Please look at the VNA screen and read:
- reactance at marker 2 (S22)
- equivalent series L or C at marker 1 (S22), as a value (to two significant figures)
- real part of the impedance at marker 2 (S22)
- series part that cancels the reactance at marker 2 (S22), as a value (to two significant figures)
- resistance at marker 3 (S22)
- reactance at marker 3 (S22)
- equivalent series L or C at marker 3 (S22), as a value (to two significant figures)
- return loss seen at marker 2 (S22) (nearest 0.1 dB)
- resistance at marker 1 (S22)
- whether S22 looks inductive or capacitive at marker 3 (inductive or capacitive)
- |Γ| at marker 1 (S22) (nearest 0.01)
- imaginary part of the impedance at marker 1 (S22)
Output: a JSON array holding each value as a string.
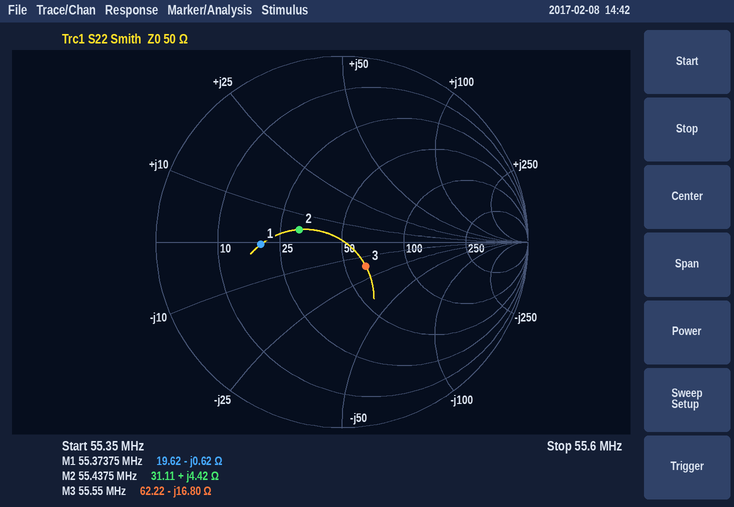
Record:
["+4.42 Ω", "4.6 nF", "31.11 Ω", "650 pF", "62.22 Ω", "-16.80 Ω", "170 pF", "12.4 dB", "19.62 Ω", "capacitive", "0.44", "-0.62 Ω"]
